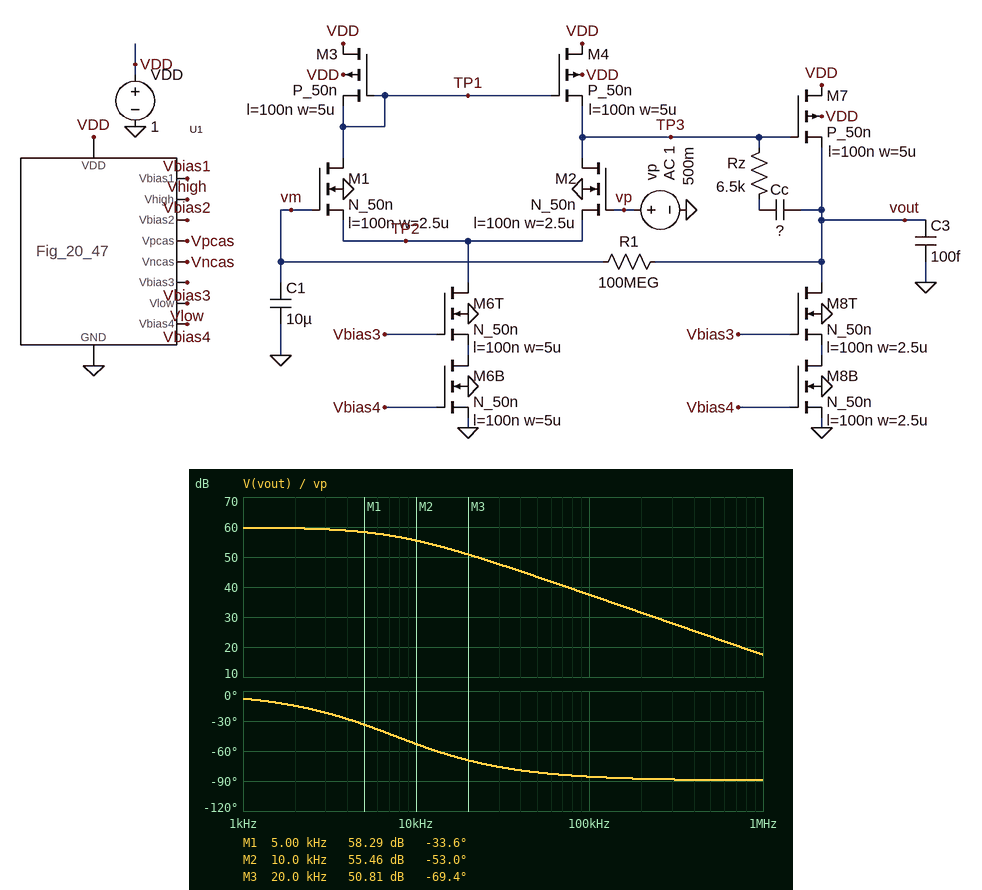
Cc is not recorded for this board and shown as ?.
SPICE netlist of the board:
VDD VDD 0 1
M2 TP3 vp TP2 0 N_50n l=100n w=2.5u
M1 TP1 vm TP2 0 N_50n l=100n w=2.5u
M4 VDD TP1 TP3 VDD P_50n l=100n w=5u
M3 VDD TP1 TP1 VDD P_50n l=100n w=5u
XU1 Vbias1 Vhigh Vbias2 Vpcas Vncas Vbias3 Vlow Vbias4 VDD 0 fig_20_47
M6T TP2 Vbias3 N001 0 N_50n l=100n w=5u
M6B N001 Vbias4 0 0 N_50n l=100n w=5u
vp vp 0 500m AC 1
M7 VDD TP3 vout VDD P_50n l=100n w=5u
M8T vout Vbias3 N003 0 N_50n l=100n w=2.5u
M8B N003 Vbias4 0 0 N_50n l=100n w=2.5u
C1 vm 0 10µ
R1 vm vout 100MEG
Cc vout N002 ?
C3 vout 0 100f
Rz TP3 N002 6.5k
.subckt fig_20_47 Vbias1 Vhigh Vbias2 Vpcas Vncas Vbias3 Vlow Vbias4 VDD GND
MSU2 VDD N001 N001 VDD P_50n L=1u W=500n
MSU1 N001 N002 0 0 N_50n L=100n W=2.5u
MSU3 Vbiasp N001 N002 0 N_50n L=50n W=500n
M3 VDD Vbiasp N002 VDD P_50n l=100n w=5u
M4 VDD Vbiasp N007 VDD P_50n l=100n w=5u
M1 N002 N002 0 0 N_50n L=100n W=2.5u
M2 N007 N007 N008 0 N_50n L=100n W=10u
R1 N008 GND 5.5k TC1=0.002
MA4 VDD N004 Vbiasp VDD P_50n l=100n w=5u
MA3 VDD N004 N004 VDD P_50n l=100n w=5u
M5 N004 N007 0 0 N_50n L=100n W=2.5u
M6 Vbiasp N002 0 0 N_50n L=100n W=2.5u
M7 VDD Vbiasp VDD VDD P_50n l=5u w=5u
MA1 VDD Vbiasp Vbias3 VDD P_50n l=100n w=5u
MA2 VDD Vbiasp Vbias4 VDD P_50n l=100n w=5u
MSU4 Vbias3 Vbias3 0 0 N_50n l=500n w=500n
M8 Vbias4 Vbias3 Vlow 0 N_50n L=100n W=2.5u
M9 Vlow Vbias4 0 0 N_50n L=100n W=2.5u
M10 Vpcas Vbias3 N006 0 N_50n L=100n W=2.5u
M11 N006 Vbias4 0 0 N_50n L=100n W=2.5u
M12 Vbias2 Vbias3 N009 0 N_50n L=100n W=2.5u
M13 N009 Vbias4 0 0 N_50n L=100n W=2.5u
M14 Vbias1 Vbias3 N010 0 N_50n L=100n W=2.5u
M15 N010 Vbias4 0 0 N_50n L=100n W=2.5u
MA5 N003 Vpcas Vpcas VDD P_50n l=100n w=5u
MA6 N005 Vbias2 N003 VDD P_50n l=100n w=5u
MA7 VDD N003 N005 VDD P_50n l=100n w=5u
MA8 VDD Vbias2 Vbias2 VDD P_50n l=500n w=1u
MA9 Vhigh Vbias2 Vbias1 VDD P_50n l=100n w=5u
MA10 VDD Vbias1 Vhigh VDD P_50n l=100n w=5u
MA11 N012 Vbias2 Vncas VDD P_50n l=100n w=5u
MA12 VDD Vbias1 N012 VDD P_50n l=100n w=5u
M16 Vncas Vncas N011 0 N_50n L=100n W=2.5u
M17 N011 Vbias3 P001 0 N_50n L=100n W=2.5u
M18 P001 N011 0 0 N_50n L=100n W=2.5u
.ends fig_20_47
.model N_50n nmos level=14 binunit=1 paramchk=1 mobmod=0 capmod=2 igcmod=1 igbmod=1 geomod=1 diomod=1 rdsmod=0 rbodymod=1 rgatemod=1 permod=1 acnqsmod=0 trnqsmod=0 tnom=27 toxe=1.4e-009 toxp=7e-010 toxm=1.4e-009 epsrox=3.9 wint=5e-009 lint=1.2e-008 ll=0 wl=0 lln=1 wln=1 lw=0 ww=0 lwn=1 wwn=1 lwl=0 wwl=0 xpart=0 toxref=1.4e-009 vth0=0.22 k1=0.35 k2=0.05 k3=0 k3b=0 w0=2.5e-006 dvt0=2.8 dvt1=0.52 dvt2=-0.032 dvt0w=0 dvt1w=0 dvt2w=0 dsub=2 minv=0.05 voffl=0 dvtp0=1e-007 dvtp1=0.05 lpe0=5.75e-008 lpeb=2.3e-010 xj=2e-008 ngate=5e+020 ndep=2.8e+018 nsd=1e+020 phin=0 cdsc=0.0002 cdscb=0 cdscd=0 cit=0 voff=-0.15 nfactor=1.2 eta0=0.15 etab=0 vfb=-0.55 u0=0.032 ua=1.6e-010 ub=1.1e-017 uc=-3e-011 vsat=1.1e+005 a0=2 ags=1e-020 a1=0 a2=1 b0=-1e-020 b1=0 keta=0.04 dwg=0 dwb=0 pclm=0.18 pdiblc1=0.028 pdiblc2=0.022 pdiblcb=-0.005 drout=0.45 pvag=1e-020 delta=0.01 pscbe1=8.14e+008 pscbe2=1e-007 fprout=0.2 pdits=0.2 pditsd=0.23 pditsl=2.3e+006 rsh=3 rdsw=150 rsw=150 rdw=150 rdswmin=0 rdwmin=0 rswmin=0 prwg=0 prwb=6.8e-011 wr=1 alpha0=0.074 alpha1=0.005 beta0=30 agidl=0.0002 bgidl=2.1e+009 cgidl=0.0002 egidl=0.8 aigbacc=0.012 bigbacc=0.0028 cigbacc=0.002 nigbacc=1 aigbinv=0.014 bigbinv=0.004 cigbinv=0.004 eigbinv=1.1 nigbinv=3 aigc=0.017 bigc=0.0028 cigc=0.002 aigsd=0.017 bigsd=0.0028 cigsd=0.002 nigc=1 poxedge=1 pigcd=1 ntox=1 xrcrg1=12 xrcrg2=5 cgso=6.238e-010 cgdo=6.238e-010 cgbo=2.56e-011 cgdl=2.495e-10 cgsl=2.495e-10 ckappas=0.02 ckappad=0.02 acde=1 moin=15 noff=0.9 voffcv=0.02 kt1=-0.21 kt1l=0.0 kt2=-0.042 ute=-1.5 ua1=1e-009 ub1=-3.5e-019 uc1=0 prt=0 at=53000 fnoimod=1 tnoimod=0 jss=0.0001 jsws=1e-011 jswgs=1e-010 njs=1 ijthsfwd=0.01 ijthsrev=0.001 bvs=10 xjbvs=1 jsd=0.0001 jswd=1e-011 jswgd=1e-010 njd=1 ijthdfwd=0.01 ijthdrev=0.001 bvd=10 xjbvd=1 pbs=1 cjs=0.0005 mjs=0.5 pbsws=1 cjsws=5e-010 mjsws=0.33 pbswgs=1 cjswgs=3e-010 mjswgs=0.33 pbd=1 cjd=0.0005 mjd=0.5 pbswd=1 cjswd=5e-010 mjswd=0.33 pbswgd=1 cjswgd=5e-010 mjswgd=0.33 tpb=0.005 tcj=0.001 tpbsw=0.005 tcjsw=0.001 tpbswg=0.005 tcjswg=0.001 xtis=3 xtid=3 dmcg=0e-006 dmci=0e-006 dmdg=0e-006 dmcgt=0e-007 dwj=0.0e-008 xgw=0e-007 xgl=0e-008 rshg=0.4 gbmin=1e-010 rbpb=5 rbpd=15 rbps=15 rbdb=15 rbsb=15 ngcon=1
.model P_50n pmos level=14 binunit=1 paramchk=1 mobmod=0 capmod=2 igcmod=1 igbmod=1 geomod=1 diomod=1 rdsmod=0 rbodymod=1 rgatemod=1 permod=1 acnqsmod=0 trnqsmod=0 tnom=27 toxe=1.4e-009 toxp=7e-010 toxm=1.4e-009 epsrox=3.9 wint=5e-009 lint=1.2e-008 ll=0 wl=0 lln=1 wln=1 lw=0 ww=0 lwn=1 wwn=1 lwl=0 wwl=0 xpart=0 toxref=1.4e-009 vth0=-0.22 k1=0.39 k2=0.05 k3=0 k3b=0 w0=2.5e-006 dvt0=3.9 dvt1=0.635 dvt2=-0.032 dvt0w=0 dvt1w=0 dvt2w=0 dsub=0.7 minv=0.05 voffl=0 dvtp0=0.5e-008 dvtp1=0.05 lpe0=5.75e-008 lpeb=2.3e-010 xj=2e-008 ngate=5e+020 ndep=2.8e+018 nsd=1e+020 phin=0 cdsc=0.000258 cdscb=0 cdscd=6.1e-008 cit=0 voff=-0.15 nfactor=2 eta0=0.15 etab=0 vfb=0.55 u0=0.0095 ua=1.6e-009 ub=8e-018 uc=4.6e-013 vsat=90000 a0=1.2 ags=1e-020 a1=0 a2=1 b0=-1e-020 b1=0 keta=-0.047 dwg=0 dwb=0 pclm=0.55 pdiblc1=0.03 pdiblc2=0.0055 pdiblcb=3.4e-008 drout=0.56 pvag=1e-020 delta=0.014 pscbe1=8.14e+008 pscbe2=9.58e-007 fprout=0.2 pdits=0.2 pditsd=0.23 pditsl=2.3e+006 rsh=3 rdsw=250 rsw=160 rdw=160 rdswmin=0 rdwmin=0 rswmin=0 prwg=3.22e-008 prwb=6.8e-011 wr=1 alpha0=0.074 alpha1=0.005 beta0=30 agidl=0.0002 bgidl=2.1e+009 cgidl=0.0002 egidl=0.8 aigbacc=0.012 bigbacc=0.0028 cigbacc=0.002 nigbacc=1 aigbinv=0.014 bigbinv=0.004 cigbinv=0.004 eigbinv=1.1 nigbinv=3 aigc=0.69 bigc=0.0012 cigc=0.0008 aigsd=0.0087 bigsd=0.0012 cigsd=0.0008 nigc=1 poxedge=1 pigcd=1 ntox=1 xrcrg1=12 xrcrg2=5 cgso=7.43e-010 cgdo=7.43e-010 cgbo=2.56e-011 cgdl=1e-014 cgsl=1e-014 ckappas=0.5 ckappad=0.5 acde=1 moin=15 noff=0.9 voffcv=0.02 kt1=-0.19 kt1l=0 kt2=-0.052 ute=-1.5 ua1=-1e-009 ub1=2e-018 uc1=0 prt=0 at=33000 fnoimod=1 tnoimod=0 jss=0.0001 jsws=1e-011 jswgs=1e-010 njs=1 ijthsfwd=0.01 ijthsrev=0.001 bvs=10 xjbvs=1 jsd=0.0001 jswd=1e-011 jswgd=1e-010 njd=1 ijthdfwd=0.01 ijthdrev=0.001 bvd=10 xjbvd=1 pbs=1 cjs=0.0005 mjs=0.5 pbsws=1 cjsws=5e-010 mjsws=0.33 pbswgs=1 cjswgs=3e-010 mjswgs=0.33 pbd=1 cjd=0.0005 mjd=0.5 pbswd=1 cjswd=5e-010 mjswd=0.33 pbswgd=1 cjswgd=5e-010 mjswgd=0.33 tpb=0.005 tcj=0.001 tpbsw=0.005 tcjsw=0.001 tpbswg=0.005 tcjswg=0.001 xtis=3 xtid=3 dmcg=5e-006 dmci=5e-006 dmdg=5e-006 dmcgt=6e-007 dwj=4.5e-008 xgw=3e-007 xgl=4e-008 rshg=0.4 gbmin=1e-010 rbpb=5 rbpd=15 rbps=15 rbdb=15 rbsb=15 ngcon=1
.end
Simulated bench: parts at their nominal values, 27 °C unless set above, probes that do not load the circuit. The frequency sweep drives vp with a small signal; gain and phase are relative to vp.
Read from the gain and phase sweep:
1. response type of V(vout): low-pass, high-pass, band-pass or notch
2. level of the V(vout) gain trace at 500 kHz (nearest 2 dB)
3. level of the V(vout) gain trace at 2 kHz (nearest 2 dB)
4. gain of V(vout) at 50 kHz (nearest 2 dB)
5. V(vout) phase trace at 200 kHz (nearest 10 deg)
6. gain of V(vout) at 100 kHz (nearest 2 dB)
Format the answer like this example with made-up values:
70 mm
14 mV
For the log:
low-pass
24 dB
60 dB
44 dB
-90 deg
38 dB
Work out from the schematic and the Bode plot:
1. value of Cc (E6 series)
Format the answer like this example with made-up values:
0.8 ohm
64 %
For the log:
3.3 pF
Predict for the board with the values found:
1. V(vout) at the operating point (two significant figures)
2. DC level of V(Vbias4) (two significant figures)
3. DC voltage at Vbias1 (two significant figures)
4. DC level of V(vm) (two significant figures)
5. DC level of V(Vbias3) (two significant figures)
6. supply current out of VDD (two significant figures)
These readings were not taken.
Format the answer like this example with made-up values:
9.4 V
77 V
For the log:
520 mV
360 mV
640 mV
500 mV
540 mV
140 µA
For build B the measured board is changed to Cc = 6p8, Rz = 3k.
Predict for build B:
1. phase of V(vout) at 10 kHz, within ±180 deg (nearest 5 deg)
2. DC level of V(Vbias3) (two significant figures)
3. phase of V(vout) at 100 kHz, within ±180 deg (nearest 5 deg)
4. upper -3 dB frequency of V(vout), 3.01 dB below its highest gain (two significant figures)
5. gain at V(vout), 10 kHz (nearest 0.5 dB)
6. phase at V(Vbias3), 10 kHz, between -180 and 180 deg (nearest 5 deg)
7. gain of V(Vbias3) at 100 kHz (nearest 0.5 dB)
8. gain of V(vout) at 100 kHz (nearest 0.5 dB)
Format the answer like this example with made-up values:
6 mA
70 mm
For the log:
-70 deg
540 mV
-90 deg
3.7 kHz
50.5 dB
0 deg
-58.5 dB
31.0 dB
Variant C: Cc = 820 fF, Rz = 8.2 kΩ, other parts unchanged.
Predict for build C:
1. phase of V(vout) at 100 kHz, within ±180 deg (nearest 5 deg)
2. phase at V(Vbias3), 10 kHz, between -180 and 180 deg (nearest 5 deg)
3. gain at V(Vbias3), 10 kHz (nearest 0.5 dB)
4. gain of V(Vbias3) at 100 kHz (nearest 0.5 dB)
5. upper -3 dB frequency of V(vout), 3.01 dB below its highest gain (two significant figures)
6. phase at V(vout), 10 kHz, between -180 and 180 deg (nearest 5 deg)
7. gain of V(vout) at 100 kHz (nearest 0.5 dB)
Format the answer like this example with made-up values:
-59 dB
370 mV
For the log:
-75 deg
50 deg
-50.0 dB
-41.0 dB
30 kHz
-20 deg
49.0 dB
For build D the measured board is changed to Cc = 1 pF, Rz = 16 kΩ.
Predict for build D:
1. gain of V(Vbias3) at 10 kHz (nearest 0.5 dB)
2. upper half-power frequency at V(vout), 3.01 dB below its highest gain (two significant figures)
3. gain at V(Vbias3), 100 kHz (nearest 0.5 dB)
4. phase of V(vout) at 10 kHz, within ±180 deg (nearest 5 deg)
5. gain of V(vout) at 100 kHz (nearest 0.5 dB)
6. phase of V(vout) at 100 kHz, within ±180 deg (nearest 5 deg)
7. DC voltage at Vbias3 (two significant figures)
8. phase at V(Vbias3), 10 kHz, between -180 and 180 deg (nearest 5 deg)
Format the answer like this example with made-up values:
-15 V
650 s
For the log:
-50.0 dB
25 kHz
-42.5 dB
-20 deg
47.5 dB
-75 deg
540 mV
45 deg
